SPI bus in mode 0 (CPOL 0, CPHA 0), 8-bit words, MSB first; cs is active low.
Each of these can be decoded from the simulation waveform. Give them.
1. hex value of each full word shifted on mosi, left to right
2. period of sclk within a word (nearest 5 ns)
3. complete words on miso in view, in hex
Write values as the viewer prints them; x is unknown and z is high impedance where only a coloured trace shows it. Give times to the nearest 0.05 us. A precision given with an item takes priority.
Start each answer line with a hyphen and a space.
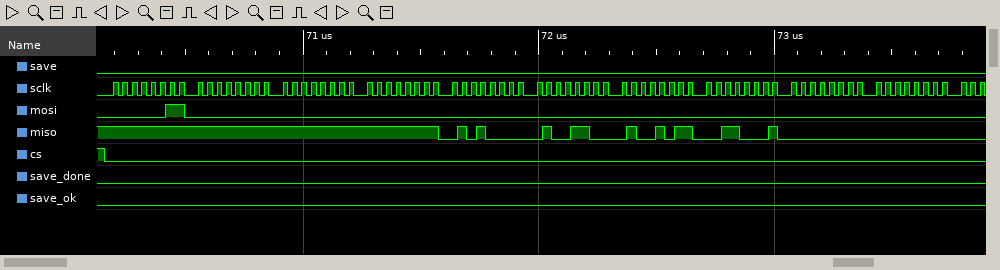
- 03, 00, 00, 00, 00, 00, 00, 00, 00, 00
- 40 ns
- FF, FF, FF, FF, 50, 4C, 4B, 31, 00, 00
